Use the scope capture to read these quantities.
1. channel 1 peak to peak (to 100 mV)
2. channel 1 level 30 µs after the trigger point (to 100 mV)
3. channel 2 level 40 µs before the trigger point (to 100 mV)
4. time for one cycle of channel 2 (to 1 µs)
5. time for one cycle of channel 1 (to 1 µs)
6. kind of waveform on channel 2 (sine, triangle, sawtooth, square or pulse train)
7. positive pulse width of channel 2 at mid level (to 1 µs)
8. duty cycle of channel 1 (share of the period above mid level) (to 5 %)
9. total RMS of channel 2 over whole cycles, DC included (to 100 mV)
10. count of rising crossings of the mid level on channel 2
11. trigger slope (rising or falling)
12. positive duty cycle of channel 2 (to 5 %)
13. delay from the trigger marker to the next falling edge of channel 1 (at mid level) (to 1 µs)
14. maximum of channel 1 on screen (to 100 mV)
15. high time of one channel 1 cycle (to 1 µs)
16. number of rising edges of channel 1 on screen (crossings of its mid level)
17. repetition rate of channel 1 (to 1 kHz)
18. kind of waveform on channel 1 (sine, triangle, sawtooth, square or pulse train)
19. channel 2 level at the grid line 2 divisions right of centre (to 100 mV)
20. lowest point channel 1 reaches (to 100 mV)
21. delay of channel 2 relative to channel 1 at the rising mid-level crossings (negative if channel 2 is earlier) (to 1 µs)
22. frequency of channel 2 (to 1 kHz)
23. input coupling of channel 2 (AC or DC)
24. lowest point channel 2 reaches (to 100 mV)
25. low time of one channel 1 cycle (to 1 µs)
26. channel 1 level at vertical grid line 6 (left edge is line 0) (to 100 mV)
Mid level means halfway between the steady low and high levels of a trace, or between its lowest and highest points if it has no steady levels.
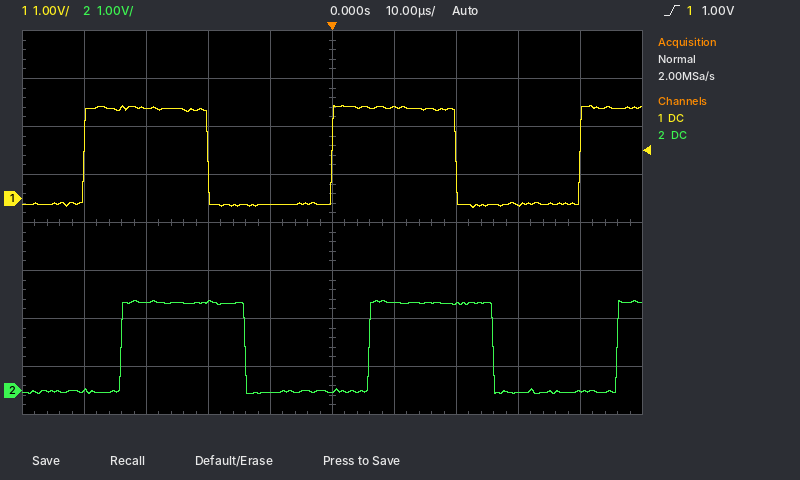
2.1 V
-100 mV
0.0 V
40 µs
40 µs
square
20 µs
50 %
1.3 V
3
rising
50 %
20 µs
1.9 V
20 µs
3
25 kHz
square
1.8 V
-200 mV
+6 µs
25 kHz
DC
-100 mV
20 µs
1.9 V
